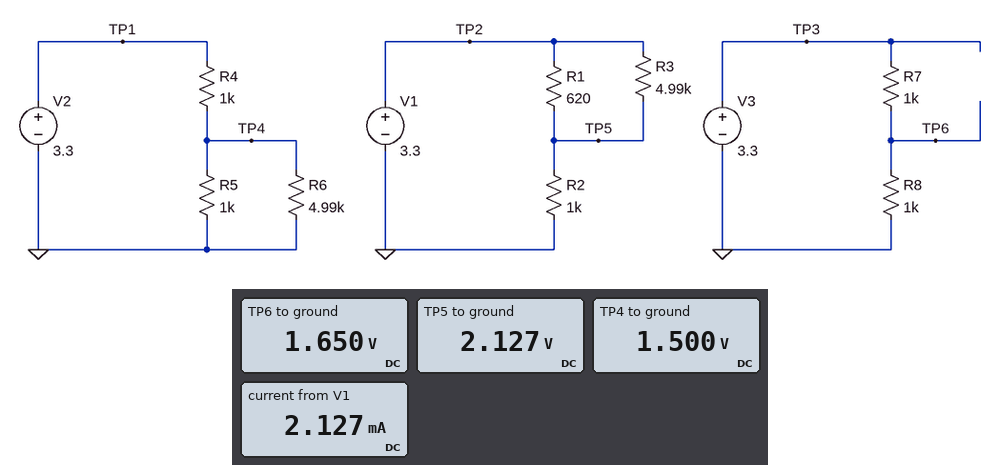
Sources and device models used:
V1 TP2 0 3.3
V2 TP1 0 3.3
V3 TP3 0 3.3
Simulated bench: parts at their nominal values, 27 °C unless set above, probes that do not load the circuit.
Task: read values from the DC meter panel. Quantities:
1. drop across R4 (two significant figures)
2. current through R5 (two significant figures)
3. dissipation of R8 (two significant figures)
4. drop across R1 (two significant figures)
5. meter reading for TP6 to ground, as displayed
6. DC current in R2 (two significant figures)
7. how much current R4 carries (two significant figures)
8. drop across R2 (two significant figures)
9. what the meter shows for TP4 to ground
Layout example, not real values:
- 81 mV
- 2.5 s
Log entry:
- 1.8 V
- 1.5 mA
- 2.7 mW
- 1.2 V
- 1.650 V
- 2.1 mA
- 1.8 mA
- 2.1 V
- 1.500 V
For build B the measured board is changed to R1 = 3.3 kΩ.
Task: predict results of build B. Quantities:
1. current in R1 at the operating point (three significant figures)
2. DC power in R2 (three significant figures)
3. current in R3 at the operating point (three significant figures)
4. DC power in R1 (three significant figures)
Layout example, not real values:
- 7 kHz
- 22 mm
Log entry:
- 665 µA
- 1.22 mW
- 440 µA
- 1.46 mW
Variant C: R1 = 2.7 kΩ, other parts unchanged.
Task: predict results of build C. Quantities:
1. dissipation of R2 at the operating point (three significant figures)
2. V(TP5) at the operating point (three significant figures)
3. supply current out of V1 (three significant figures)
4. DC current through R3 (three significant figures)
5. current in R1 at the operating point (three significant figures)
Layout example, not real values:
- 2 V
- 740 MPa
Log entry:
- 1.44 mW
- 1.20 V
- 1.20 mA
- 421 µA
- 778 µA
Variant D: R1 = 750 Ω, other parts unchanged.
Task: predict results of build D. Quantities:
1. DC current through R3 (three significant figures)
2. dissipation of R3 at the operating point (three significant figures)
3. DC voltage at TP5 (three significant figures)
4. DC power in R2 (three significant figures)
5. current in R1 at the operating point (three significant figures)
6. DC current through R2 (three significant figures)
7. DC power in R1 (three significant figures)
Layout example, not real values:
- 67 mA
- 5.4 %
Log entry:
- 261 µA
- 340 µW
- 2.00 V
- 3.99 mW
- 1.74 mA
- 2.00 mA
- 2.26 mW
